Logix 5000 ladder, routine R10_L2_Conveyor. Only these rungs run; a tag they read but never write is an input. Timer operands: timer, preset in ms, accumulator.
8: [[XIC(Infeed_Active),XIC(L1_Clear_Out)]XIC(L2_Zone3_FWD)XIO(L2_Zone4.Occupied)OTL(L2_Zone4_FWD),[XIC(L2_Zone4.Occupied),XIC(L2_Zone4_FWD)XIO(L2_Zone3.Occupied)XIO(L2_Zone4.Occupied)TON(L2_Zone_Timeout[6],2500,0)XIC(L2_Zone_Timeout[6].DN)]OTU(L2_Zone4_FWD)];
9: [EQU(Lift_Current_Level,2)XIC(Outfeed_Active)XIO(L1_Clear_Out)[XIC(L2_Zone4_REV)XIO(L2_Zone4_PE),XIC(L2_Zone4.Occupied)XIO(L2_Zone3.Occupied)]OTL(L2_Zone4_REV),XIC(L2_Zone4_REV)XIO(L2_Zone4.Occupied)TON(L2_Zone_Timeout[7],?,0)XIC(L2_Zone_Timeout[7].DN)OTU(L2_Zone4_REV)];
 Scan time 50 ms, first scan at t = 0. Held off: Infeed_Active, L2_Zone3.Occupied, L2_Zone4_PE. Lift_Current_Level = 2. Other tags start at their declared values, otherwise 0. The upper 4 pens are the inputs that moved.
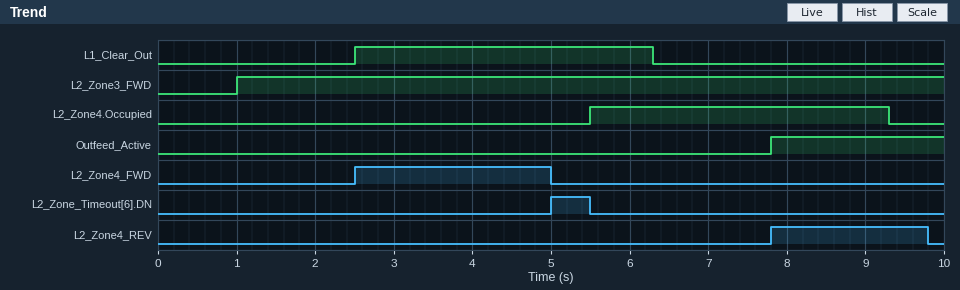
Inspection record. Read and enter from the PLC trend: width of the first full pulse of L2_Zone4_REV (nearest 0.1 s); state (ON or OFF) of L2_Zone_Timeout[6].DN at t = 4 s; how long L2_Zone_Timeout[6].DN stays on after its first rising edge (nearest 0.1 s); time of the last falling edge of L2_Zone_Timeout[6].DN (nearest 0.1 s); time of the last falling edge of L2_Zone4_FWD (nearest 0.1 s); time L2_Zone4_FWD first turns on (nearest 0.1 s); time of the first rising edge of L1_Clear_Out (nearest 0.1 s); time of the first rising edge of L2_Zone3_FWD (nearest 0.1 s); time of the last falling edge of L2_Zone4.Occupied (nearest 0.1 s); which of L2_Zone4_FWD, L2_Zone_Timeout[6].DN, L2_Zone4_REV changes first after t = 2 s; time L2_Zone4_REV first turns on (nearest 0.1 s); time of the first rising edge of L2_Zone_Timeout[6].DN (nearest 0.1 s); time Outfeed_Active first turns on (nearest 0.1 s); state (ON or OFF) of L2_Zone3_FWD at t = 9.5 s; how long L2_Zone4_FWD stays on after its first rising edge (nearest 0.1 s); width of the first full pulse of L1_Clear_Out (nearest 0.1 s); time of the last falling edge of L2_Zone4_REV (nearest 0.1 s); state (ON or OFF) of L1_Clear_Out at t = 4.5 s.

2.0 s
OFF
0.5 s
5.5 s
5.0 s
2.5 s
2.5 s
1.0 s
9.3 s
L2_Zone4_FWD
7.8 s
5.0 s
7.8 s
ON
2.5 s
3.8 s
9.8 s
ON
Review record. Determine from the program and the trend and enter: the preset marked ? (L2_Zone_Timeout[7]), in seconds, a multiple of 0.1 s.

0.5 s
